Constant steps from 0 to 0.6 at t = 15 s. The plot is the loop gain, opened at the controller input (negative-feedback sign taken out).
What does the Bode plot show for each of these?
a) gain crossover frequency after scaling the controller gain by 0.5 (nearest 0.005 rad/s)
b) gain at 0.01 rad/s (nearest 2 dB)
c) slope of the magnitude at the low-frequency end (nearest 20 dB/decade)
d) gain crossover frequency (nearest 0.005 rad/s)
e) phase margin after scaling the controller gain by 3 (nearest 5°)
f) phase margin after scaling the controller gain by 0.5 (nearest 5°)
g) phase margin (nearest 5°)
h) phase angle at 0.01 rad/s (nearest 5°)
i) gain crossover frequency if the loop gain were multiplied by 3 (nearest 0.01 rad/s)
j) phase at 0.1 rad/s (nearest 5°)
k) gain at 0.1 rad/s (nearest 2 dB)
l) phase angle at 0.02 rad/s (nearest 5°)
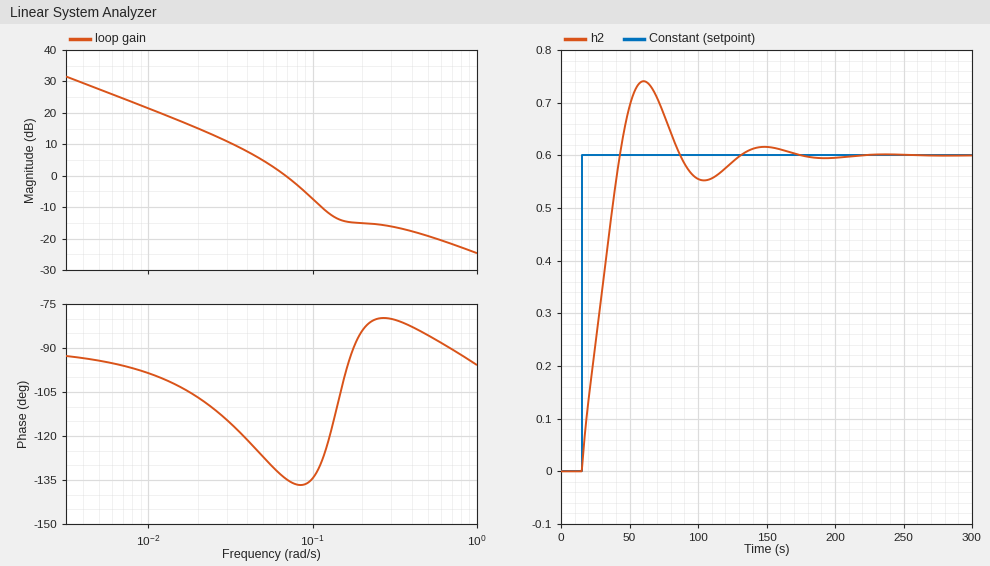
0.045 rad/s
22 dB
-20 dB/decade
0.070 rad/s
50°
55°
45°
-100°
0.11 rad/s
-135°
-8 dB
-105°
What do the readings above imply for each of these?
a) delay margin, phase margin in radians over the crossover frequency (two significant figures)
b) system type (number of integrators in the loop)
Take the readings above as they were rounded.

11 s
1
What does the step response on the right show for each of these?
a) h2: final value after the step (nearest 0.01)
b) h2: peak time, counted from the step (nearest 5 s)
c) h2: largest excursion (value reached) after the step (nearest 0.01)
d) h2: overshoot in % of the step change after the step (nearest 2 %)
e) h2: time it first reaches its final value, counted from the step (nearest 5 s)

0.60
45 s
0.74
24 %
30 s
